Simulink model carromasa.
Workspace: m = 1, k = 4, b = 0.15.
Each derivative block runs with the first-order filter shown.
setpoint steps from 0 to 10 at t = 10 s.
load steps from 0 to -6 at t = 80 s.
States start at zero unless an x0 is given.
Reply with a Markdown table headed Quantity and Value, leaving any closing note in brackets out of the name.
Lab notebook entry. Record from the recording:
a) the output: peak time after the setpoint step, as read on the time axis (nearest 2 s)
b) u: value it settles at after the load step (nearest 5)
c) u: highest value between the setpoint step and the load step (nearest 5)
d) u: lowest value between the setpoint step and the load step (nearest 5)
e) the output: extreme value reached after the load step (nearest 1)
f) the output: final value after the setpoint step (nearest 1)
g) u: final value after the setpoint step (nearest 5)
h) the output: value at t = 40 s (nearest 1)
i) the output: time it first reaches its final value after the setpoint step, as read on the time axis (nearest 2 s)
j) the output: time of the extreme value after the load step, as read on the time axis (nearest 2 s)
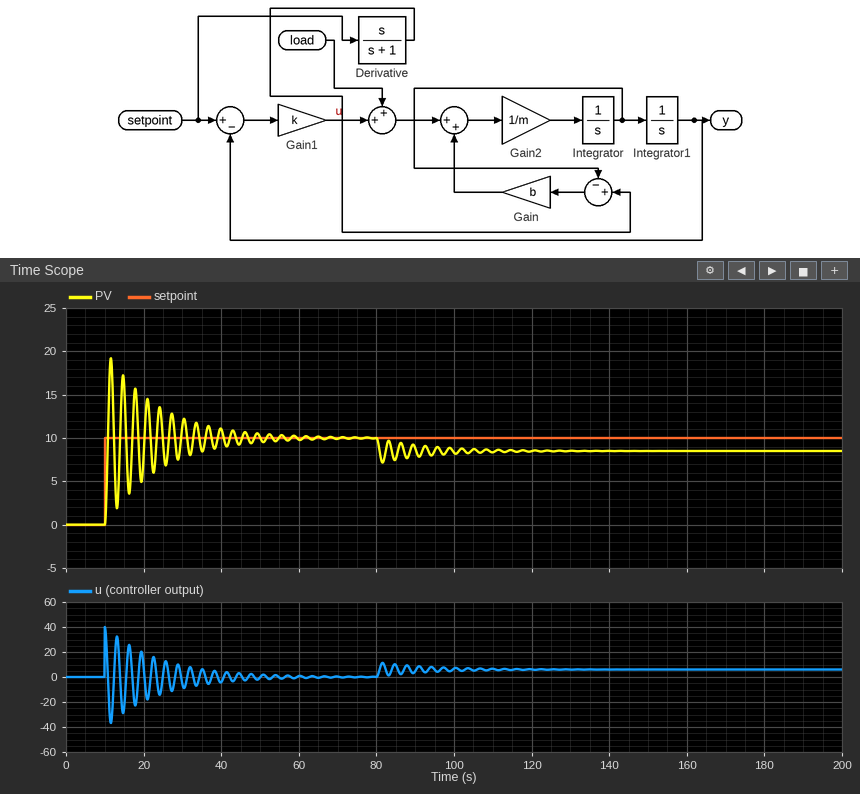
| Quantity | Value |
|---|---|
| the output: peak time after the setpoint step, as read on the time axis | 12 s |
| u: value it settles at after the load step | 5 |
| u: highest value between the setpoint step and the load step | 40 |
| u: lowest value between the setpoint step and the load step | -35 |
| the output: extreme value reached after the load step | 7 |
| the output: final value after the setpoint step | 10 |
| u: final value after the setpoint step | 0 |
| the output: value at t = 40 s | 11 |
| the output: time it first reaches its final value after the setpoint step, as read on the time axis | 10 s |
| the output: time of the extreme value after the load step, as read on the time axis | 82 s |
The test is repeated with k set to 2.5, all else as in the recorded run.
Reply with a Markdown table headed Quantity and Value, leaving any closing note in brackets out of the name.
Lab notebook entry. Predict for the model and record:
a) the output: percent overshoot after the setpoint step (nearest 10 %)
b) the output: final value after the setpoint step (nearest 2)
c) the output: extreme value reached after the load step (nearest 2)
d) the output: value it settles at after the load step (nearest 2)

| Quantity | Value |
|---|---|
| the output: percent overshoot after the setpoint step | 90 % |
| the output: final value after the setpoint step | 10 |
| the output: extreme value reached after the load step | 6 |
| the output: value it settles at after the load step | 8 |
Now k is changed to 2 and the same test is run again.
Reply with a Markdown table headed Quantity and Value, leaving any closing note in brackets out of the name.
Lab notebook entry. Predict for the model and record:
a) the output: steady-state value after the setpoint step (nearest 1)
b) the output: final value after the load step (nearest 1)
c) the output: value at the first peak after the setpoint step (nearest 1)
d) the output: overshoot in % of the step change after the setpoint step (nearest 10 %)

| Quantity | Value |
|---|---|
| the output: steady-state value after the setpoint step | 10 |
| the output: final value after the load step | 7 |
| the output: value at the first peak after the setpoint step | 19 |
| the output: overshoot in % of the step change after the setpoint step | 90 % |
